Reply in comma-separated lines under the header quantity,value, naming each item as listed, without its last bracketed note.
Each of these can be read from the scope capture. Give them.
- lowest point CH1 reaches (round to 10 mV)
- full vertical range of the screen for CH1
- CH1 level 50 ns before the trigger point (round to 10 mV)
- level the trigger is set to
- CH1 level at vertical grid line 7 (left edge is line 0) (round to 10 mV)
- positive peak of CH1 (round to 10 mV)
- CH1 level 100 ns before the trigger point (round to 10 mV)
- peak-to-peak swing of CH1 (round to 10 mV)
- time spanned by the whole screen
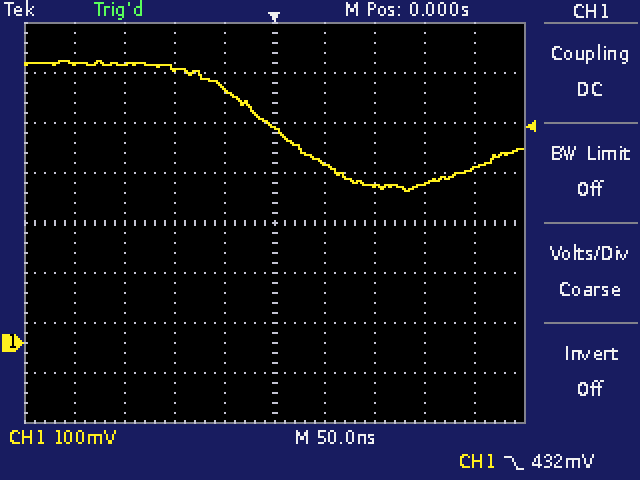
quantity,value
lowest point CH1 reaches,300 mV
full vertical range of the screen for CH1,800 mV
CH1 level 50 ns before the trigger point,510 mV
level the trigger is set to,432 mV
CH1 level at vertical grid line 7 (left edge is line 0),310 mV
positive peak of CH1,560 mV
CH1 level 100 ns before the trigger point,550 mV
peak-to-peak swing of CH1,260 mV
time spanned by the whole screen,500 ns
